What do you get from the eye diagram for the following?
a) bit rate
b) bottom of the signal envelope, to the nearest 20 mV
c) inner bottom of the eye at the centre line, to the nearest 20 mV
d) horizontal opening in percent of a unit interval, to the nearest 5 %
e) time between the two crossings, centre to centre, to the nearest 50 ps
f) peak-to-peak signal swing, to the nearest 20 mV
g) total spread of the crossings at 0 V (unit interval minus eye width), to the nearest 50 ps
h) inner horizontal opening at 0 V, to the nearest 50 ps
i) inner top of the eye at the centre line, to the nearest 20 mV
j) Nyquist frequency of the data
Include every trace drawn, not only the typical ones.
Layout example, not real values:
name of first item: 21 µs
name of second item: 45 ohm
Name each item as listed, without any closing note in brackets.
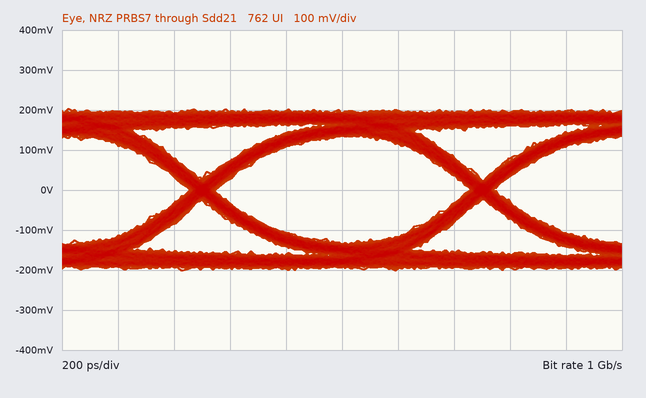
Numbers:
bit rate: 1 Gb/s
bottom of the signal envelope, to the nearest 20 mV: -200 mV
inner bottom of the eye at the centre line, to the nearest 20 mV: -140 mV
horizontal opening in percent of a unit interval, to the nearest 5 %: 90 %
time between the two crossings, centre to centre, to the nearest 50 ps: 1.00 ns
peak-to-peak signal swing, to the nearest 20 mV: 400 mV
total spread of the crossings at 0 V (unit interval minus eye width), to the nearest 50 ps: 100 ps
inner horizontal opening at 0 V, to the nearest 50 ps: 900 ps
inner top of the eye at the centre line, to the nearest 20 mV: 140 mV
Nyquist frequency of the data: 500 MHz
